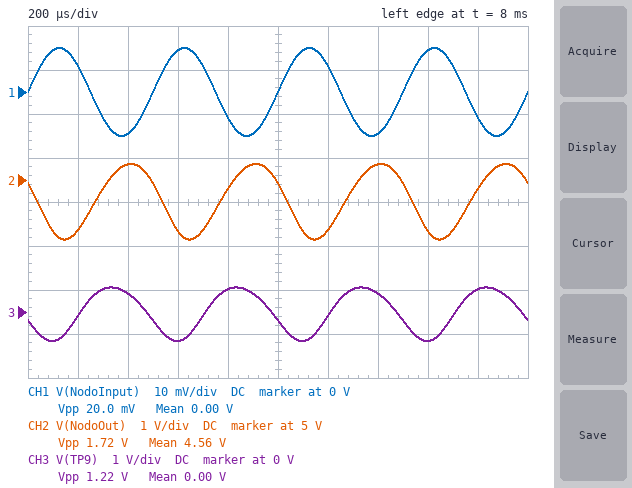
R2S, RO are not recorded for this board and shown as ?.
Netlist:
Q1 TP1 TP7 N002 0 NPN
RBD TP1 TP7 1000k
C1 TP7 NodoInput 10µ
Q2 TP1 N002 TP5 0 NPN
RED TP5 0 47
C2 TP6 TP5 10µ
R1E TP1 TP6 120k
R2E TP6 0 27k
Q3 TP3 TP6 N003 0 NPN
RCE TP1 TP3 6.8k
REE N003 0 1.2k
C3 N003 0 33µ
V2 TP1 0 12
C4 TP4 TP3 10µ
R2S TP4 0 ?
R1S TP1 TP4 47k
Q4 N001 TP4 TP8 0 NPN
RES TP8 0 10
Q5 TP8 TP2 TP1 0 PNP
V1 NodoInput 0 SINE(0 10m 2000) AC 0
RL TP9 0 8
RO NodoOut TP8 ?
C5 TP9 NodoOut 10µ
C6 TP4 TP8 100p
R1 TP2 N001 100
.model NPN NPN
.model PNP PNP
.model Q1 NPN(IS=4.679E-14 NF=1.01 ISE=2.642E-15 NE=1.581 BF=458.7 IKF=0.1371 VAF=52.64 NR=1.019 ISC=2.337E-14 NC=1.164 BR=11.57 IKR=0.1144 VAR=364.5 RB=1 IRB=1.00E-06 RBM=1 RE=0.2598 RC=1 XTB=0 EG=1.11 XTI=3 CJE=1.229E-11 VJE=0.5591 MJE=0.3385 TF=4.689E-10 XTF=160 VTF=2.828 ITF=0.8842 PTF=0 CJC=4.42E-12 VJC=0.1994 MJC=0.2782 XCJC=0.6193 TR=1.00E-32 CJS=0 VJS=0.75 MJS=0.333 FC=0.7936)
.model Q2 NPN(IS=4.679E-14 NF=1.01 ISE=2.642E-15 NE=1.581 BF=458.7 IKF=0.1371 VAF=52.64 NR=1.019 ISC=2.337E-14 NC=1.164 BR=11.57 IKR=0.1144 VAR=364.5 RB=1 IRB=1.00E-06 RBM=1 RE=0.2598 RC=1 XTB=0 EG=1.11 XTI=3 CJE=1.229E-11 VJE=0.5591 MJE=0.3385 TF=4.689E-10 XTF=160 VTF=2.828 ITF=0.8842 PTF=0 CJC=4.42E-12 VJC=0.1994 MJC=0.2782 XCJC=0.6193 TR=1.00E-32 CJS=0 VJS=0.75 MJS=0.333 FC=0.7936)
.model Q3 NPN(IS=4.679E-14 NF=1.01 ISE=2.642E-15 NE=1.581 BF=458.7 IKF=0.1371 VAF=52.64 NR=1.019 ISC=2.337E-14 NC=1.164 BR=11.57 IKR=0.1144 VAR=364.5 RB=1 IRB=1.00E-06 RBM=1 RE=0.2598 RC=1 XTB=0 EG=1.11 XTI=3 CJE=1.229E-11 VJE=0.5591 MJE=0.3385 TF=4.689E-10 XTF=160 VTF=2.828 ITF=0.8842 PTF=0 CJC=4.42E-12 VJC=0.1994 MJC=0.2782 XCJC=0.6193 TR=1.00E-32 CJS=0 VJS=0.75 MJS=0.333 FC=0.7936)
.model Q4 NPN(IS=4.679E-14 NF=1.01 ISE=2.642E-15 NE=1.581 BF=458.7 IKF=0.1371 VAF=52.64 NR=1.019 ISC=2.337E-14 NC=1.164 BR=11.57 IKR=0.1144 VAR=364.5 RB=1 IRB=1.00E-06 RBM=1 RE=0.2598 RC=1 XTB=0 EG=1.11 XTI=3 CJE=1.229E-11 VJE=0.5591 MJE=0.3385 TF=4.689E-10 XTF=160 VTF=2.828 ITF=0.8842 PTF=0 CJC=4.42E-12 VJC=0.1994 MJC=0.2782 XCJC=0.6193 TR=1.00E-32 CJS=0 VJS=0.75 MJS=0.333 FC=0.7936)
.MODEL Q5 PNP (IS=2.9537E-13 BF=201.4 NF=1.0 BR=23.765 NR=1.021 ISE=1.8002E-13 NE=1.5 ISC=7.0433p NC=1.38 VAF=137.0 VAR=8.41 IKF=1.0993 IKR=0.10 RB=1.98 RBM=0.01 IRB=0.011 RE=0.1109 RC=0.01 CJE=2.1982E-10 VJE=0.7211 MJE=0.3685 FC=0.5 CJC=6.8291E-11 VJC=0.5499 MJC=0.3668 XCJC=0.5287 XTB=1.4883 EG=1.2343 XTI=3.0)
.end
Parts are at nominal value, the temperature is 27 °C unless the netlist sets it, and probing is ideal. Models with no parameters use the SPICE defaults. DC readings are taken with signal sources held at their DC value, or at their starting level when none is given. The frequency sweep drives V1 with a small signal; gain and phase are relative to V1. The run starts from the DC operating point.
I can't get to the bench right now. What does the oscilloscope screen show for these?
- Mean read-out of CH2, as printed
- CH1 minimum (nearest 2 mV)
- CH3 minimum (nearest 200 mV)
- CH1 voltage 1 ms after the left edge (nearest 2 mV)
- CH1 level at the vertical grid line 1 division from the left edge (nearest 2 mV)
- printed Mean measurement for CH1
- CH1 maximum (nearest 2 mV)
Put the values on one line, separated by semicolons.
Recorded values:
4.56 V; -10 mV; -600 mV; 0 V; 6 mV; 0.00 V; 10 mV
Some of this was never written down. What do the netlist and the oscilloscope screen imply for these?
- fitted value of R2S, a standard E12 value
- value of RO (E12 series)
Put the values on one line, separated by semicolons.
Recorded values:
56 kΩ; 15 Ω
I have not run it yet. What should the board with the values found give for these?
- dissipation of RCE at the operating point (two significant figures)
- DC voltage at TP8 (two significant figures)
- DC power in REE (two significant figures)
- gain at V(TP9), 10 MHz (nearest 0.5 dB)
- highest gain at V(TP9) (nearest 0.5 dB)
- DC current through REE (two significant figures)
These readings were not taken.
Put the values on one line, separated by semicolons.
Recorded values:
6.8 mW; 4.6 V; 1.2 mW; 36.0 dB; 36.5 dB; 1.0 mA
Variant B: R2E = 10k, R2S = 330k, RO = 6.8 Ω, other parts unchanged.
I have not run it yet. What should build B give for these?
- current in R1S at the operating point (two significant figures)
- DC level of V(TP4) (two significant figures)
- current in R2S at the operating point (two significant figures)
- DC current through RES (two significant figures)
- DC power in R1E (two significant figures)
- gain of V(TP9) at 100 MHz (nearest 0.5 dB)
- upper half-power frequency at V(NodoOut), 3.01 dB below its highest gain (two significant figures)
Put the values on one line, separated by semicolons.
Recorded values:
91 µA; 7.7 V; 23 µA; 690 mA; 1.0 mW; 17.0 dB; 1.7 kHz
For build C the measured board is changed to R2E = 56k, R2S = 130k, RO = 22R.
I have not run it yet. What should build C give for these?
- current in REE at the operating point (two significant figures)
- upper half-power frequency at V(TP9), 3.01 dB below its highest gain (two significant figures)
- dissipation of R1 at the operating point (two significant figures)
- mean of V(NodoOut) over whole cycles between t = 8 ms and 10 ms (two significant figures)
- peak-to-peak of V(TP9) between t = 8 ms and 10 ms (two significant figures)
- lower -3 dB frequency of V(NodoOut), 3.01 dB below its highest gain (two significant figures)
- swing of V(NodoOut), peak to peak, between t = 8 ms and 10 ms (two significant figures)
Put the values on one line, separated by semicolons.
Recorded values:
1.5 mA; 410 MHz; 3.5 mW; 7.0 V; 860 mV; 240 Hz; 1.3 V
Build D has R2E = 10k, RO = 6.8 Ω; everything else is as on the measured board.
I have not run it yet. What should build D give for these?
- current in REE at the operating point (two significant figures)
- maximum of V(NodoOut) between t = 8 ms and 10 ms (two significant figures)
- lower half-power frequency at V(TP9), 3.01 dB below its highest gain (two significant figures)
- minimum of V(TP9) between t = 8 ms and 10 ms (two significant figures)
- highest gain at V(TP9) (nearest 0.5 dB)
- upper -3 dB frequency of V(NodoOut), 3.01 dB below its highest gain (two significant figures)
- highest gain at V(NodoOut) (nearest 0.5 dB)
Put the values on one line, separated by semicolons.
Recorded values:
150 µA; 4.7 V; 1.0 kHz; -150 mV; 23.5 dB; 1.7 kHz; 29.0 dB
